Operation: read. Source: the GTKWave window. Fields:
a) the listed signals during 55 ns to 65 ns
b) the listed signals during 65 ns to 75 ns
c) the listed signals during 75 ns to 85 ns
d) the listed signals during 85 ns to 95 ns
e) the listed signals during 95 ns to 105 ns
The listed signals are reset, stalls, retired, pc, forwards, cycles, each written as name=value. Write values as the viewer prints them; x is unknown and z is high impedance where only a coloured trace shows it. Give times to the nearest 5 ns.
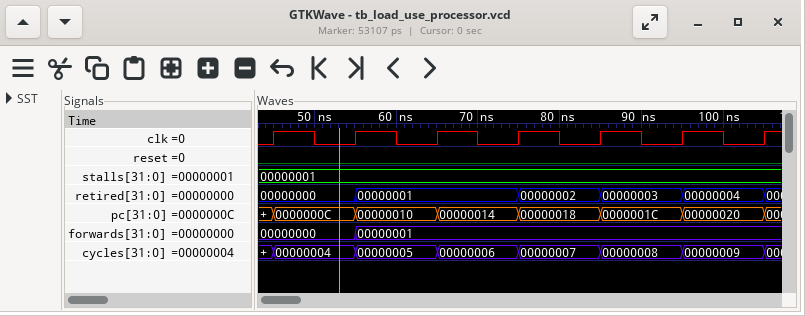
reset=0, stalls=00000001, retired=00000001, pc=00000010, forwards=00000001, cycles=00000005
reset=0, stalls=00000001, retired=00000001, pc=00000014, forwards=00000001, cycles=00000006
reset=0, stalls=00000001, retired=00000002, pc=00000018, forwards=00000001, cycles=00000007
reset=0, stalls=00000001, retired=00000003, pc=0000001C, forwards=00000001, cycles=00000008
reset=0, stalls=00000001, retired=00000004, pc=00000020, forwards=00000001, cycles=00000009
